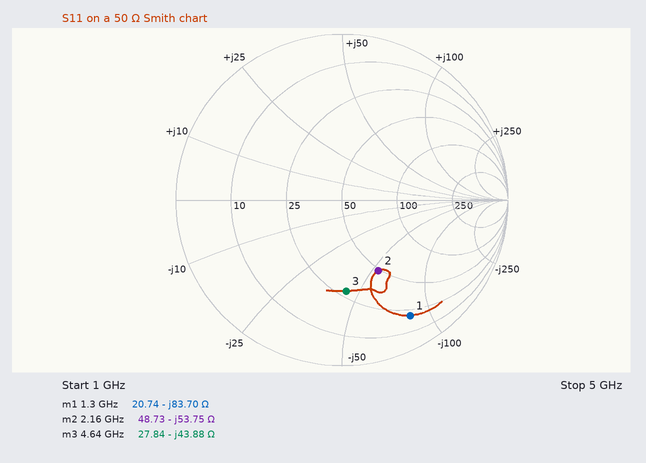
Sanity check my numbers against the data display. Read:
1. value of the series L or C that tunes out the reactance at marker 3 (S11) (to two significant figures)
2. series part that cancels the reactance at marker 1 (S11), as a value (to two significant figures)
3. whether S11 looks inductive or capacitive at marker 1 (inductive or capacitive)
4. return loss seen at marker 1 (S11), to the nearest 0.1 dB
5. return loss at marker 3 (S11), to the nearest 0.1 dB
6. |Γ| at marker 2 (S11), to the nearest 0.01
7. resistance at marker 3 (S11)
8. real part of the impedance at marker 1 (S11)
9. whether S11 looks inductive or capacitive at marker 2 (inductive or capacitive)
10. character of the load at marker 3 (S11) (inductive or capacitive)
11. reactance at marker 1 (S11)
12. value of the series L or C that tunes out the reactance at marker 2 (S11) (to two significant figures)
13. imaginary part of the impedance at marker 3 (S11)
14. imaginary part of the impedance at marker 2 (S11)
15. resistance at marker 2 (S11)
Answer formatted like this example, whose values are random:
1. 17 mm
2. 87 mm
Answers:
1. 1.5 nH
2. 10 nH
3. capacitive
4. 1.8 dB
5. 5.2 dB
6. 0.48
7. 27.84 Ω
8. 20.74 Ω
9. capacitive
10. capacitive
11. -83.70 Ω
12. 4.0 nH
13. -43.88 Ω
14. -53.75 Ω
15. 48.73 Ω
